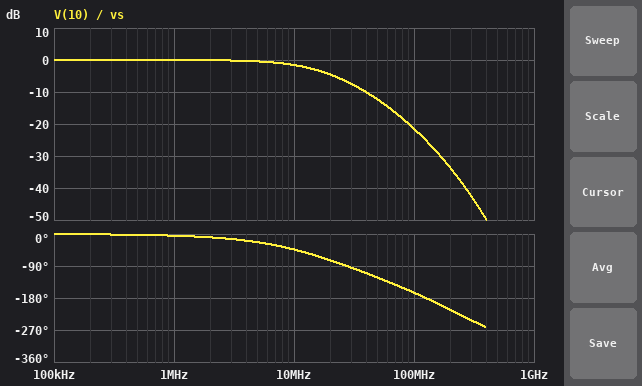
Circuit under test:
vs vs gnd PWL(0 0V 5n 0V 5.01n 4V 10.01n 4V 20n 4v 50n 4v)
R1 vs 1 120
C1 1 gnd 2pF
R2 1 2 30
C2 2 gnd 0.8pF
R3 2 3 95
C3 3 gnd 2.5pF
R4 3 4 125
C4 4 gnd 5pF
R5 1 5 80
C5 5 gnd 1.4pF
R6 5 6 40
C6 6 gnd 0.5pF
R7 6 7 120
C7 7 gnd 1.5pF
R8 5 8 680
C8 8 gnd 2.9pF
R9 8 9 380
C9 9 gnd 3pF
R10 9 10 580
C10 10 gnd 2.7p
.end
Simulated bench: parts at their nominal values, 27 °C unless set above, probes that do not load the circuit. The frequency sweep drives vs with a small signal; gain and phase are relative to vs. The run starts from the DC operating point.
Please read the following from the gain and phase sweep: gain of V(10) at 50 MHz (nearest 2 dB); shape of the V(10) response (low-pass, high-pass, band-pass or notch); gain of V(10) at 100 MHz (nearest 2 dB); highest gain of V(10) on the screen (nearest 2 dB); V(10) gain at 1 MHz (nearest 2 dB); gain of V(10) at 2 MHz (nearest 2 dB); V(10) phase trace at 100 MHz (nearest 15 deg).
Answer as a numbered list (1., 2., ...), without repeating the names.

1. -12 dB
2. low-pass
3. -22 dB
4. 0 dB
5. 0 dB
6. 0 dB
7. -165 deg
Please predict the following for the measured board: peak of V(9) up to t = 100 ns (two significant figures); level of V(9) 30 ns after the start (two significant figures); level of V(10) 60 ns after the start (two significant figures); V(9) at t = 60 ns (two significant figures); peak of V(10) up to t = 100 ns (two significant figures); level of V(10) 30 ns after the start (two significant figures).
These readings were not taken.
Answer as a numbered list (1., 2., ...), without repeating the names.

1. 4.0 V
2. 3.6 V
3. 4.0 V
4. 4.0 V
5. 4.0 V
6. 3.5 V
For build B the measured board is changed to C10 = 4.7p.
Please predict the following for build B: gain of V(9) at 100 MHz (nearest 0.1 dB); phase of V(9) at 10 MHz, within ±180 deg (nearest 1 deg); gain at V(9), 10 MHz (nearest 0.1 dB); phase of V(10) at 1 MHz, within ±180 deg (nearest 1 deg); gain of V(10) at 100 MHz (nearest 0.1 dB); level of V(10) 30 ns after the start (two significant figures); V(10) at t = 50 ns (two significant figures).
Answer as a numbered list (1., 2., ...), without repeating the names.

1. -18.9 dB
2. -43 deg
3. -2.3 dB
4. -6 deg
5. -24.8 dB
6. 3.2 V
7. 3.8 V
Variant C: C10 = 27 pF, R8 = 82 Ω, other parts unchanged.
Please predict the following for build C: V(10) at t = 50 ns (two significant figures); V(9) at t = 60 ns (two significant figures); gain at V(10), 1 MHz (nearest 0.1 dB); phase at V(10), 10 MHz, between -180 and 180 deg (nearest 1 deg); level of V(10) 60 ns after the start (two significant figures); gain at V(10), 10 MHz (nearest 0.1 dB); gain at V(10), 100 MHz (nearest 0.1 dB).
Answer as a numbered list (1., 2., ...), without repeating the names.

1. 2.8 V
2. 3.5 V
3. -0.2 dB
4. -77 deg
5. 3.1 V
6. -7.8 dB
7. -32.7 dB
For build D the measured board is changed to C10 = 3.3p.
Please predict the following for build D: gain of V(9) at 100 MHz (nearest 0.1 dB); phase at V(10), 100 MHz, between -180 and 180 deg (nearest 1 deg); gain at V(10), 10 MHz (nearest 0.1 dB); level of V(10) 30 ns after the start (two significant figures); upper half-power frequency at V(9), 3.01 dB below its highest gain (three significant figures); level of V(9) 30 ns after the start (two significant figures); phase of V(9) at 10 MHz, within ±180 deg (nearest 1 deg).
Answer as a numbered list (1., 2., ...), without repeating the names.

1. -18.7 dB
2. -169 deg
3. -1.8 dB
4. 3.4 V
5. 14.1 MHz
6. 3.5 V
7. -40 deg
